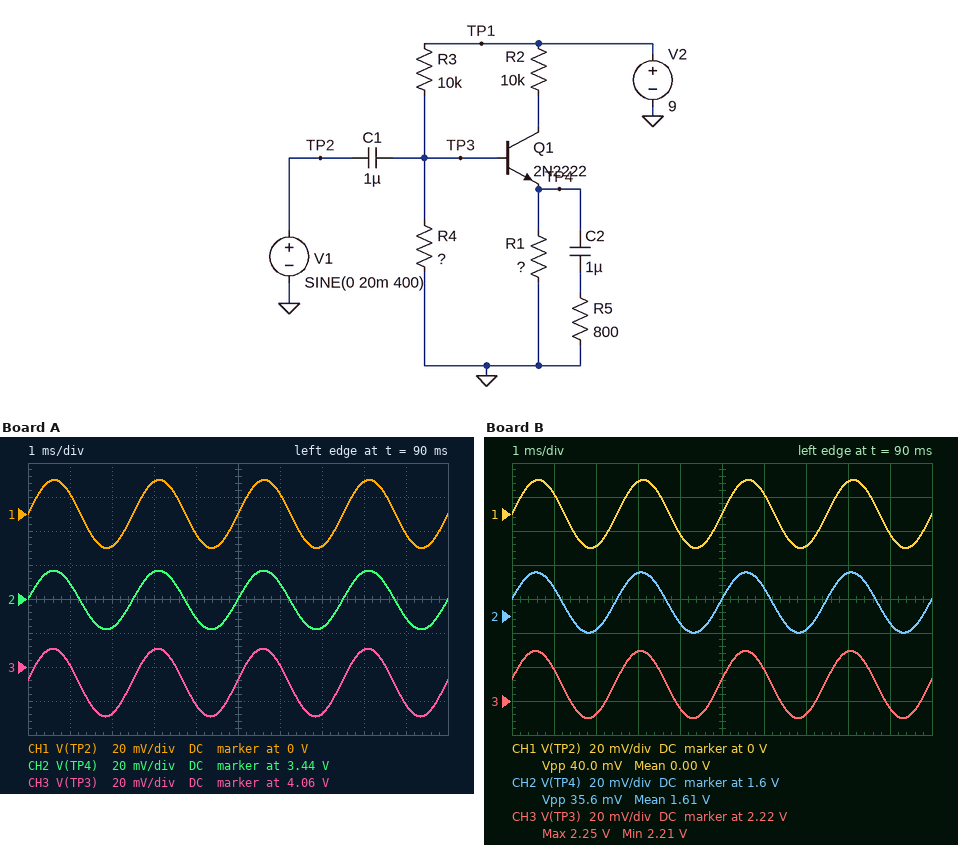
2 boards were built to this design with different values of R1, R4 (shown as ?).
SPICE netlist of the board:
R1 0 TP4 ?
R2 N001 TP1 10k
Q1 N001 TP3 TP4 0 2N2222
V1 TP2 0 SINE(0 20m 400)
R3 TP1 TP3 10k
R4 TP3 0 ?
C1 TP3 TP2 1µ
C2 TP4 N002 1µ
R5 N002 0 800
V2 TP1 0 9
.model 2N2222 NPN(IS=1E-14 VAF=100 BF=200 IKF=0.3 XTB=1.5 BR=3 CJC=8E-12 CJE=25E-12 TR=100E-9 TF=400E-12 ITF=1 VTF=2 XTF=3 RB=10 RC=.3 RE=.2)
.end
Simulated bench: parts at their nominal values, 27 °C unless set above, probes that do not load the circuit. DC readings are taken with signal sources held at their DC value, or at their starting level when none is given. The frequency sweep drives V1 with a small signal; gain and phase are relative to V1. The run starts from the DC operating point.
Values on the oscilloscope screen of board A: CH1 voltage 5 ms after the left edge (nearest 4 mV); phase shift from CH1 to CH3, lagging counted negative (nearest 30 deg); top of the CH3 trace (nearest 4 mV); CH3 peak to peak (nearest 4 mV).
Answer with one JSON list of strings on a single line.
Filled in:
["0 V", "0 deg", "4.072 V", "40 mV"]
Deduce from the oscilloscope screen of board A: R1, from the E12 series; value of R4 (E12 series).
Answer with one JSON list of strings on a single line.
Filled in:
["18 kΩ", "8.2 kΩ"]
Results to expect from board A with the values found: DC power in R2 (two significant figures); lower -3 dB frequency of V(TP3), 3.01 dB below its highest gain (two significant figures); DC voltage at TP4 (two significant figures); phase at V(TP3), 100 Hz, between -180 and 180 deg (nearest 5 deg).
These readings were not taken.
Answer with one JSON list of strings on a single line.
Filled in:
["360 µW", "36 Hz", "3.4 V", "20 deg"]
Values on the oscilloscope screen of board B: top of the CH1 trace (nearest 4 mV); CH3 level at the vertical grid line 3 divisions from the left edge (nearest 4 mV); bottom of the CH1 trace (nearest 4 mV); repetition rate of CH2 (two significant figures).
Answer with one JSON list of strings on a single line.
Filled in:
["20 mV", "2.248 V", "-20 mV", "400 Hz"]
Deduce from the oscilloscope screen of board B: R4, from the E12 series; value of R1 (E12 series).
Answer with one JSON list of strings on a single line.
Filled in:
["3.3 kΩ", "5.6 kΩ"]
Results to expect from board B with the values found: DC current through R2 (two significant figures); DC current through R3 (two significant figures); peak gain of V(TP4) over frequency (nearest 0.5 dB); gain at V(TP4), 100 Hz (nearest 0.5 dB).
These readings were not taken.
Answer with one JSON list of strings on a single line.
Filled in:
["290 µA", "680 µA", "-1.0 dB", "-2.0 dB"]
